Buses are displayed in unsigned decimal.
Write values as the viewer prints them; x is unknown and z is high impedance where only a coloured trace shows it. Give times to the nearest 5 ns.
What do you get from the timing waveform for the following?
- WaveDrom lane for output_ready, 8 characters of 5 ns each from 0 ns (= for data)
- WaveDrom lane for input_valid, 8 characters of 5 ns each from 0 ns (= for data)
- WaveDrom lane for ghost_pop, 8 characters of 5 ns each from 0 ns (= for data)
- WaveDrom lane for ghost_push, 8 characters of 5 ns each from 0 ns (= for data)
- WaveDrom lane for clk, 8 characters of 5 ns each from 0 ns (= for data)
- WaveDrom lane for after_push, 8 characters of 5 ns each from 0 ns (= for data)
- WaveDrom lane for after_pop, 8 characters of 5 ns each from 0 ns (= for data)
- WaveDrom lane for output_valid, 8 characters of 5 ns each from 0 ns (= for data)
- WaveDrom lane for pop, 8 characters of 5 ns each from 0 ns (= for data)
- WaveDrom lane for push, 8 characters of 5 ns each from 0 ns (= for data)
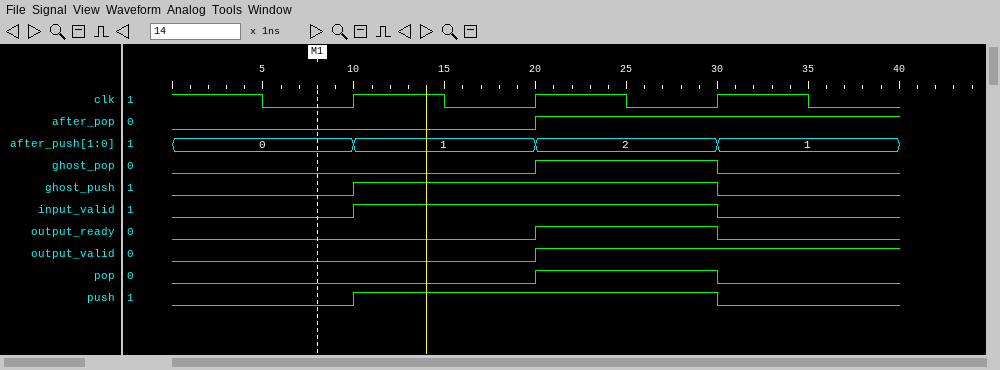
{name: 'output_ready', wave: '0...1.0.'}
{name: 'input_valid', wave: '0.1...0.'}
{name: 'ghost_pop', wave: '0...1.0.'}
{name: 'ghost_push', wave: '0.1...0.'}
{name: 'clk', wave: '10101010'}
{name: 'after_push', wave: '=.=.=.=.', data: '0 1 2 1'}
{name: 'after_pop', wave: '0...1...'}
{name: 'output_valid', wave: '0...1...'}
{name: 'pop', wave: '0...1.0.'}
{name: 'push', wave: '0.1...0.'}
